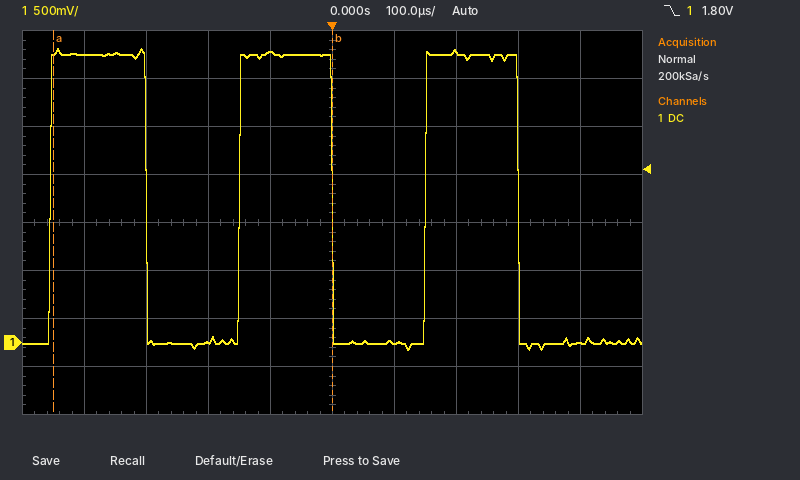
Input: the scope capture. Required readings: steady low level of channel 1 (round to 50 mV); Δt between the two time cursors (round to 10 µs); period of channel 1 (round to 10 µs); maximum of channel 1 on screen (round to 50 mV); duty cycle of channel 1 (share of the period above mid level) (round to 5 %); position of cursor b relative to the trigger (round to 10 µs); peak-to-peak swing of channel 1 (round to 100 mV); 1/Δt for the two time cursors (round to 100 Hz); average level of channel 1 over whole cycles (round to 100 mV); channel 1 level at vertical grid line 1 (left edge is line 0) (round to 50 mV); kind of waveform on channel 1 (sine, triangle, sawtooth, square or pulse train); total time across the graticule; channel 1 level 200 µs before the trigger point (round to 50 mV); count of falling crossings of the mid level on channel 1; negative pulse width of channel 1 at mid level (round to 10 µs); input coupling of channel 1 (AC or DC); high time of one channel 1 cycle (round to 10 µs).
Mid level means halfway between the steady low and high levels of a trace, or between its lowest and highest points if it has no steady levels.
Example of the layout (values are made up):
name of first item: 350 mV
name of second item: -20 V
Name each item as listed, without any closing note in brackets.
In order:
steady low level of channel 1: 0 mV
Δt between the two time cursors: 450 µs
period of channel 1: 300 µs
maximum of channel 1 on screen: 3.05 V
duty cycle of channel 1 (share of the period above mid level): 50 %
position of cursor b relative to the trigger: 0 µs
peak-to-peak swing of channel 1: 3.10 V
1/Δt for the two time cursors: 2.2 kHz
average level of channel 1 over whole cycles: 1.5 V
channel 1 level at vertical grid line 1 (left edge is line 0): 3.00 V
kind of waveform on channel 1: square
total time across the graticule: 1 ms
channel 1 level 200 µs before the trigger point: 0 mV
count of falling crossings of the mid level on channel 1: 3
negative pulse width of channel 1 at mid level: 150 µs
input coupling of channel 1: DC
high time of one channel 1 cycle: 150 µs
